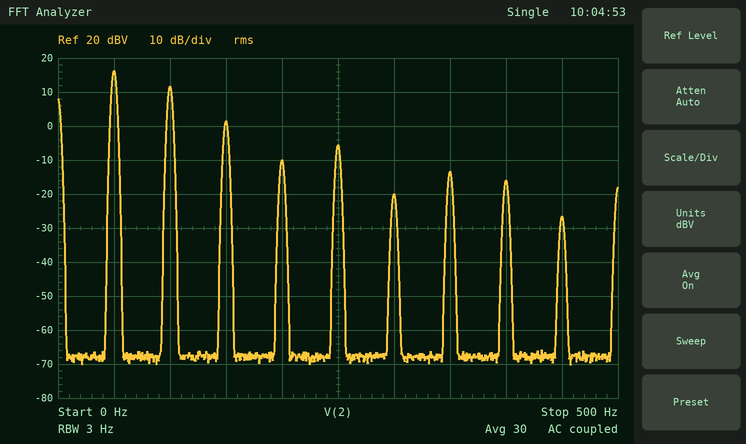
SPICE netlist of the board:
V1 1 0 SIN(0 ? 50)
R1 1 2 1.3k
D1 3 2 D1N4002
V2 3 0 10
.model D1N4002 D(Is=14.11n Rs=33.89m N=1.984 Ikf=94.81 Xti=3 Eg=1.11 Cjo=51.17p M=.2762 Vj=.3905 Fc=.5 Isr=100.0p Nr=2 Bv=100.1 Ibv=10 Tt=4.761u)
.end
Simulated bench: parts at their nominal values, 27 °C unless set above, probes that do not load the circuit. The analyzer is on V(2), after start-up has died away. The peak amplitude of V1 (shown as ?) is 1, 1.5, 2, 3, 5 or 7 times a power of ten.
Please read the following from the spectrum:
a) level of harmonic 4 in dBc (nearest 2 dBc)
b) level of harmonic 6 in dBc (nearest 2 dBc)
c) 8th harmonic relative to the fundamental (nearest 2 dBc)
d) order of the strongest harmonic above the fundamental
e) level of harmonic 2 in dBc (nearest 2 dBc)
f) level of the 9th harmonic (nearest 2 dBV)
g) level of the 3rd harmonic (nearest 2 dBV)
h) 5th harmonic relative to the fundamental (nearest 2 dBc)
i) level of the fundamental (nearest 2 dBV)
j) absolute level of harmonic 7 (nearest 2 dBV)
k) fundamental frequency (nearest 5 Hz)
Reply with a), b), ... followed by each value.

a) -26 dBc
b) -36 dBc
c) -32 dBc
d) 2
e) -4 dBc
f) -26 dBV
g) 2 dBV
h) -22 dBc
i) 16 dBV
j) -14 dBV
k) 50 Hz
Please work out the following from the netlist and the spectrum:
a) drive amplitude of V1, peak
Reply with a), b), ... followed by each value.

a) 30 V
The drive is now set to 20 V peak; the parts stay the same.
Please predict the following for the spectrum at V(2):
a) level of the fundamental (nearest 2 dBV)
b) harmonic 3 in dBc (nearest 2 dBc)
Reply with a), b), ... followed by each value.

a) 10 dBV
b) -10 dBc
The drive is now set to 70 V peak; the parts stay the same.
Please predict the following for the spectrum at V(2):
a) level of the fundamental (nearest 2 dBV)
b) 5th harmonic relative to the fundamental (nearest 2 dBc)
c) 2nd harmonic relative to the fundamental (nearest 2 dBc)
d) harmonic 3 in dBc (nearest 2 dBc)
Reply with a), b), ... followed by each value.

a) 26 dBV
b) -28 dBc
c) -6 dBc
d) -24 dBc
